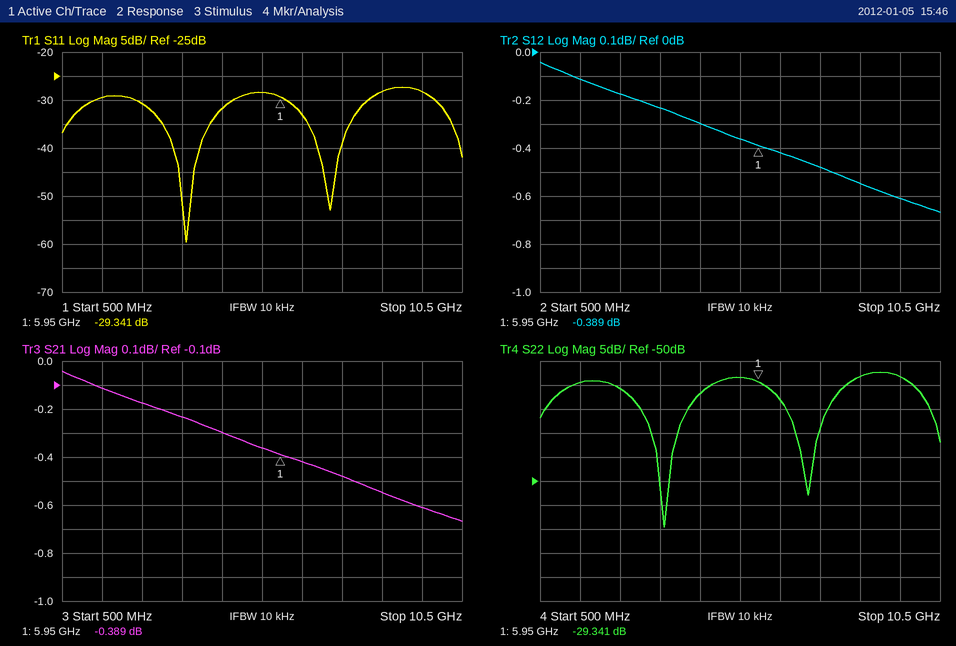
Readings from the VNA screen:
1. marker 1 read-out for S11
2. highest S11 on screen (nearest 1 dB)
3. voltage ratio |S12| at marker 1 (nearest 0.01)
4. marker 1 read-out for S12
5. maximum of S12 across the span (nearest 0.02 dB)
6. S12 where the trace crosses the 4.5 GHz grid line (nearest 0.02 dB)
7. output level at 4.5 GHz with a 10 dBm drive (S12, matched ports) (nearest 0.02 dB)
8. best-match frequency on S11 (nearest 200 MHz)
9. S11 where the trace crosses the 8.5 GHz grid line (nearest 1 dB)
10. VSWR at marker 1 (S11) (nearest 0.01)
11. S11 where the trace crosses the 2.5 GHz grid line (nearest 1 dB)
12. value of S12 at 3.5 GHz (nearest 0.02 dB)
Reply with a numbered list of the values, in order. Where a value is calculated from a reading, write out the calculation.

1. -29.341 dB
2. -27 dB
3. 10^(-0.389/20) ≈ 0.96
4. -0.389 dB
5. -0.04 dB
6. -0.30 dB
7. 10 dBm + (-0.30 dB) = 9.70 dBm
8. 3.6 GHz
9. -28 dB
10. (1 + 0.0341)/(1 − 0.0341) ≈ 1.07
11. -31 dB
12. -0.24 dB
